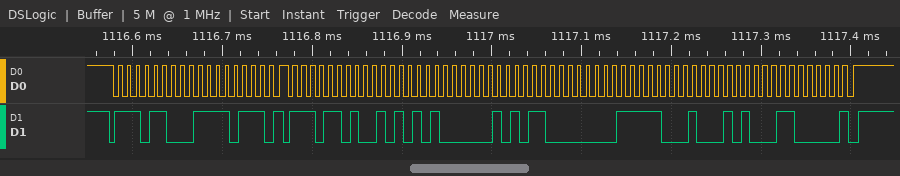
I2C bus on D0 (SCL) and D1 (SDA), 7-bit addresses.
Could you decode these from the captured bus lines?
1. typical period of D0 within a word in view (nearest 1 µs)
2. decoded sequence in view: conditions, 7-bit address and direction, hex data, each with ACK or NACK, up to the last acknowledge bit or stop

10 µs
start, address 76 write ACK, F7 ACK, repeated start, address 76 read ACK, 55 ACK, 05 ACK, C0 ACK, 7C ACK, 8A ACK, 60 NACK, stop
